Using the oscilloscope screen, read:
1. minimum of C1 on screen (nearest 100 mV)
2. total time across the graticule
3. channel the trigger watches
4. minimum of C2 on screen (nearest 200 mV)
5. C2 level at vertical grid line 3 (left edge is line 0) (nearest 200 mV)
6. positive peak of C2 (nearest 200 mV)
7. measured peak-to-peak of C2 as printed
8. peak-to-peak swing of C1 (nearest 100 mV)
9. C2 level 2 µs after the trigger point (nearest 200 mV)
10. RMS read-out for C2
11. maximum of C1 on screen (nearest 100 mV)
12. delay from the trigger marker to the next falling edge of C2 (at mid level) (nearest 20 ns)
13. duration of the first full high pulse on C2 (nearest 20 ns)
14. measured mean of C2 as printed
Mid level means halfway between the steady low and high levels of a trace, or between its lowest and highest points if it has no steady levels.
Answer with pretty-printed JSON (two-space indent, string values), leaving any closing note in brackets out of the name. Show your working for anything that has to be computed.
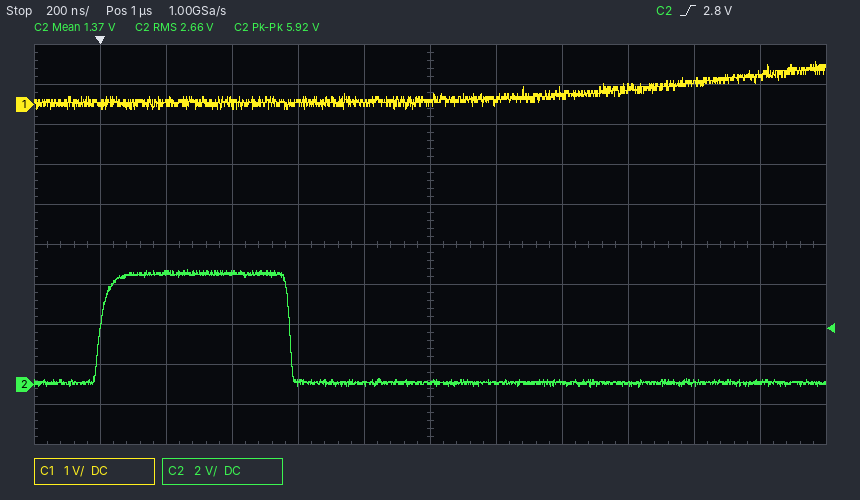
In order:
{
  "minimum of C1 on screen": "-100 mV",
  "total time across the graticule": "2.4 µs",
  "channel the trigger watches": "C2",
  "minimum of C2 on screen": "-200 mV",
  "C2 level at vertical grid line 3 (left edge is line 0)": "5.6 V",
  "positive peak of C2": "5.8 V",
  "measured peak-to-peak of C2 as printed": "5.92 V",
  "peak-to-peak swing of C1": "1.1 V − (-100 mV) = 1.2 V",
  "C2 level 2 µs after the trigger point": "200 mV",
  "RMS read-out for C2": "2.66 V",
  "maximum of C1 on screen": "1.1 V",
  "delay from the trigger marker to the next falling edge of C2 (at mid level)": "580 ns",
  "duration of the first full high pulse on C2": "580 ns",
  "measured mean of C2 as printed": "1.37 V"
}
